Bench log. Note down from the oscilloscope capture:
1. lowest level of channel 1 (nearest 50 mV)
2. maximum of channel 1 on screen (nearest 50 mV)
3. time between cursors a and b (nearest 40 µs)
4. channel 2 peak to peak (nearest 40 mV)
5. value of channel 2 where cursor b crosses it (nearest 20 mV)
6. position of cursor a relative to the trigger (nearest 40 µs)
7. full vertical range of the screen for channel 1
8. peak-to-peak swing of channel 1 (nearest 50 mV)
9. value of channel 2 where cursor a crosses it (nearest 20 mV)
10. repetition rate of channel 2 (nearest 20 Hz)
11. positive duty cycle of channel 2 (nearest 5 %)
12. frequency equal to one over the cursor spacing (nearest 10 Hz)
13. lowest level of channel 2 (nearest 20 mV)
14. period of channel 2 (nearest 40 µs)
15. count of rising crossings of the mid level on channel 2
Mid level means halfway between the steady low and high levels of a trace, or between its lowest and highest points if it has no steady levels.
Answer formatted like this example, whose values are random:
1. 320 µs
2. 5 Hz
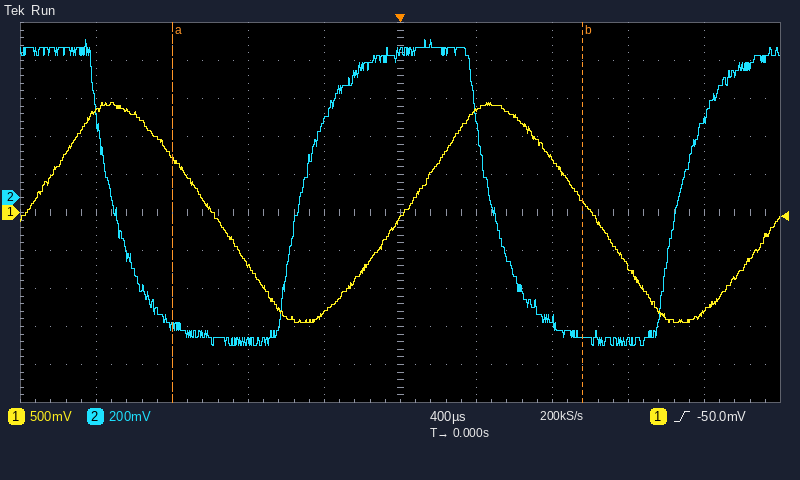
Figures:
1. -1.45 V
2. 1.45 V
3. 2.16 ms
4. 1.60 V
5. -740 mV
6. -1.20 ms
7. 5 V
8. 2.90 V
9. -680 mV
10. 500 Hz
11. 50 %
12. 460 Hz
13. -780 mV
14. 2.00 ms
15. 2
